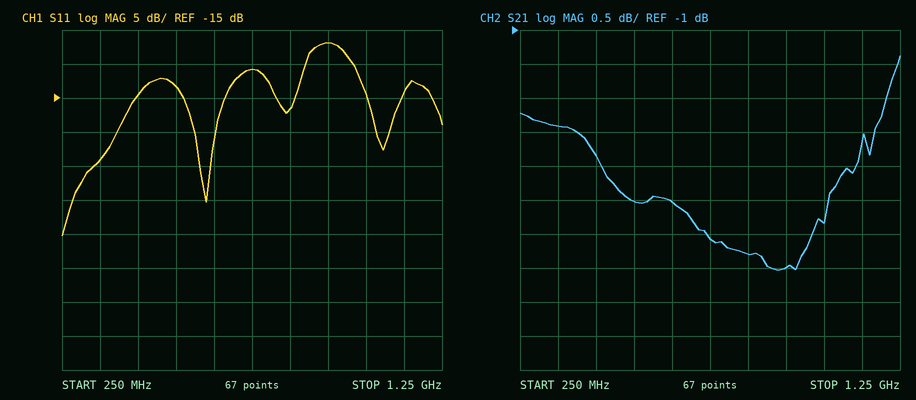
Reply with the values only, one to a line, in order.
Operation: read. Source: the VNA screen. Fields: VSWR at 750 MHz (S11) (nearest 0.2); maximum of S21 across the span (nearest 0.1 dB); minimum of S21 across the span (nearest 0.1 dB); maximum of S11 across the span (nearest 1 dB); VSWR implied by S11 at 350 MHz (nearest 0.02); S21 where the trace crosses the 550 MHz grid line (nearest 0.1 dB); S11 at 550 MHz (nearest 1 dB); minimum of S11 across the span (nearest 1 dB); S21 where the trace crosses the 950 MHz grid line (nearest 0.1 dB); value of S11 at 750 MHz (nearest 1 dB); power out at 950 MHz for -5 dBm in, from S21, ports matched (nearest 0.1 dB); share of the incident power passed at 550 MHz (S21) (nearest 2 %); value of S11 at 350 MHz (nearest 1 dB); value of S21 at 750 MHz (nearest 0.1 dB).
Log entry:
1.8
-1.4 dB
-4.5 dB
-7 dB
1.14
-3.5 dB
-13 dB
-35 dB
-4.5 dB
-11 dB
-9.5 dBm
44 %
-24 dB
-4.1 dB
